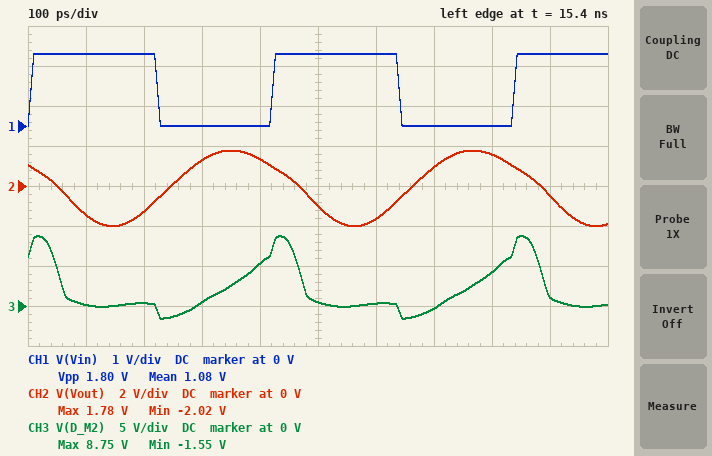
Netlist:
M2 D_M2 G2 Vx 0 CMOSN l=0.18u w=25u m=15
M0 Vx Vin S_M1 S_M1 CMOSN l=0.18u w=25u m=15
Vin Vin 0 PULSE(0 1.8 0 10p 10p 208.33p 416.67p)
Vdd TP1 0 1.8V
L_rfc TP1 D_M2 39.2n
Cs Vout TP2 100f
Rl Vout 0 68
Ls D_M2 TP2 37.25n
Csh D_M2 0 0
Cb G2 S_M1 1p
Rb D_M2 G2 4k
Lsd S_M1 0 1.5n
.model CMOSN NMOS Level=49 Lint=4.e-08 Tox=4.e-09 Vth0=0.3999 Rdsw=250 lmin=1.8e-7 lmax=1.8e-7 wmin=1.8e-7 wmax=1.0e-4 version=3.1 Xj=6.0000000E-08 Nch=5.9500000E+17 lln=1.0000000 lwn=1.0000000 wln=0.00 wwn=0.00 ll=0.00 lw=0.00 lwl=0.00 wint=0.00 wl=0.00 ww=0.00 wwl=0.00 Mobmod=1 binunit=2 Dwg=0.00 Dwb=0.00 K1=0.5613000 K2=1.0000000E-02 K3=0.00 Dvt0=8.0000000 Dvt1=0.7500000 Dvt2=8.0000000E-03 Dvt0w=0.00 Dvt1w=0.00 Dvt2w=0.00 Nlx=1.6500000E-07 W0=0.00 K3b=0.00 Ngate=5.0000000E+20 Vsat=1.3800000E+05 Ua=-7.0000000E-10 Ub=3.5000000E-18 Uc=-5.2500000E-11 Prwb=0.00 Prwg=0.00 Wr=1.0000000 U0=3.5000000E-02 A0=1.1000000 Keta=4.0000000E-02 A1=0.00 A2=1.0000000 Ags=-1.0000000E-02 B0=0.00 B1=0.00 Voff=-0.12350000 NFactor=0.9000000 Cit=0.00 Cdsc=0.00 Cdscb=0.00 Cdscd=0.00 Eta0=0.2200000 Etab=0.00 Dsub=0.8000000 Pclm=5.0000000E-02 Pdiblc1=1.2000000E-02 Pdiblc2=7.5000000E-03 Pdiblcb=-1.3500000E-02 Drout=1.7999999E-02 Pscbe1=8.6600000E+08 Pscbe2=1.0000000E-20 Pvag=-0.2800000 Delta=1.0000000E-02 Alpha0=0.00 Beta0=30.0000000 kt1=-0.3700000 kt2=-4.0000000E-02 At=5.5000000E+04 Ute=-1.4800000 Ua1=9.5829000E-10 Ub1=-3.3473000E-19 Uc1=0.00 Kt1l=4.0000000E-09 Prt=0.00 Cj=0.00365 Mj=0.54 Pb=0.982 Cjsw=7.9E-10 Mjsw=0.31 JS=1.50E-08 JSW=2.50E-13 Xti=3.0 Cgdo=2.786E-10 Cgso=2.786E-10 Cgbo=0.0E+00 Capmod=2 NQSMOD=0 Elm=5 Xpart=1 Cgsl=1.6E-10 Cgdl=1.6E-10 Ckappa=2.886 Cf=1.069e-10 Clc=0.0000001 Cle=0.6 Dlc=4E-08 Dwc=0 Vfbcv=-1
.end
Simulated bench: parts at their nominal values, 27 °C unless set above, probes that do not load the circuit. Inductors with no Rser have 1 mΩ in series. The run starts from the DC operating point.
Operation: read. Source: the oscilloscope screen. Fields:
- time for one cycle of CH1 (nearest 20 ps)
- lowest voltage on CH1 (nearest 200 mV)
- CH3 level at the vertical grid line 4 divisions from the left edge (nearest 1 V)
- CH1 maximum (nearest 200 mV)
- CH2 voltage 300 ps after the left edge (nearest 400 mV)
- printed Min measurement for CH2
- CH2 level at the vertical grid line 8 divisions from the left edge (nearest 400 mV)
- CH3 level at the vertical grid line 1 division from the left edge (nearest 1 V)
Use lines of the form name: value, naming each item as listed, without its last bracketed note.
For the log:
time for one cycle of CH1: 420 ps
lowest voltage on CH1: 0 V
CH3 level at the vertical grid line 4 divisions from the left edge: 5 V
CH1 maximum: 1.8 V
CH2 voltage 300 ps after the left edge: 1.2 V
printed Min measurement for CH2: -2.02 V
CH2 level at the vertical grid line 8 divisions from the left edge: 1.6 V
CH3 level at the vertical grid line 1 division from the left edge: 0 V
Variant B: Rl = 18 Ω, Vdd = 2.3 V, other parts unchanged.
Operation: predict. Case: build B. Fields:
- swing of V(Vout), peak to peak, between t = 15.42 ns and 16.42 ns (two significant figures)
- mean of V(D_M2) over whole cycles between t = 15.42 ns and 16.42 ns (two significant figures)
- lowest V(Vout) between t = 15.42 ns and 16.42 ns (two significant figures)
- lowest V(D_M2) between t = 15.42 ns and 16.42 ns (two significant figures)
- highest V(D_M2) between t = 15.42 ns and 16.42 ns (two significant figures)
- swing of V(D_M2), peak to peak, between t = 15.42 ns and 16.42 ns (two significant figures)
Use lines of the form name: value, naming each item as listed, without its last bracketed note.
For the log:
swing of V(Vout), peak to peak, between t = 15.42 ns and 16.42 ns: 1.7 V
mean of V(D_M2) over whole cycles between t = 15.42 ns and 16.42 ns: 2.3 V
lowest V(Vout) between t = 15.42 ns and 16.42 ns: -890 mV
lowest V(D_M2) between t = 15.42 ns and 16.42 ns: -2.3 V
highest V(D_M2) between t = 15.42 ns and 16.42 ns: 14 V
swing of V(D_M2), peak to peak, between t = 15.42 ns and 16.42 ns: 16 V
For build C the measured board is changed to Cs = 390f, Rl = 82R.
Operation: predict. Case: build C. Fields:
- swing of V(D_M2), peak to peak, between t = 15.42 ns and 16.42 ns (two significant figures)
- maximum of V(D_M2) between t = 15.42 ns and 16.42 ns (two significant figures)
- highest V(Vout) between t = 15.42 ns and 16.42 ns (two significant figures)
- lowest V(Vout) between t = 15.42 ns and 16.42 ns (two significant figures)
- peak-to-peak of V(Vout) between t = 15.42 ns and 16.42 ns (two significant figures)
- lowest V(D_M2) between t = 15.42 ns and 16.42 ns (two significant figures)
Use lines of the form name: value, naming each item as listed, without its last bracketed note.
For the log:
swing of V(D_M2), peak to peak, between t = 15.42 ns and 16.42 ns: 8.1 V
maximum of V(D_M2) between t = 15.42 ns and 16.42 ns: 7.0 V
highest V(Vout) between t = 15.42 ns and 16.42 ns: 610 mV
lowest V(Vout) between t = 15.42 ns and 16.42 ns: -560 mV
peak-to-peak of V(Vout) between t = 15.42 ns and 16.42 ns: 1.2 V
lowest V(D_M2) between t = 15.42 ns and 16.42 ns: -1.1 V
